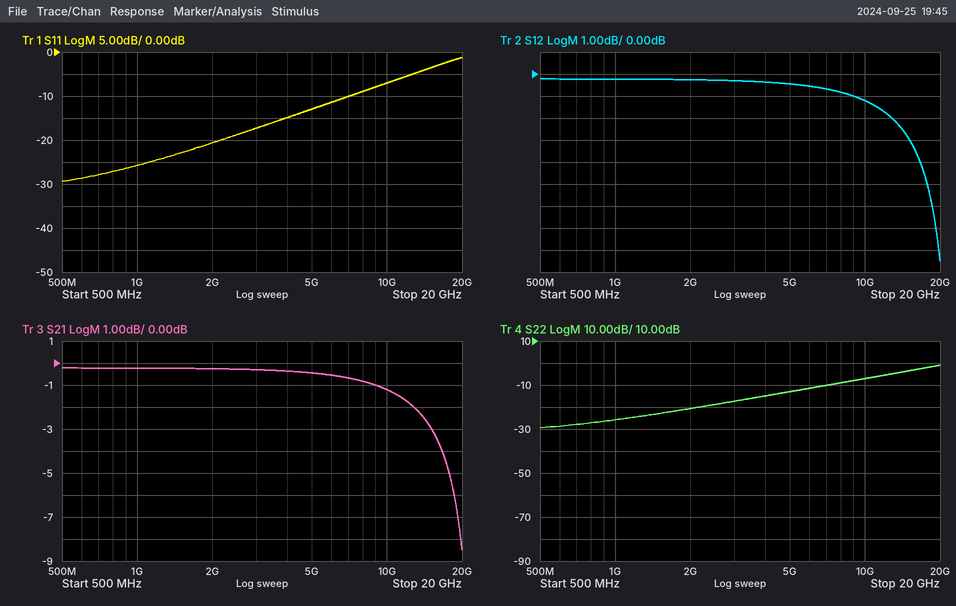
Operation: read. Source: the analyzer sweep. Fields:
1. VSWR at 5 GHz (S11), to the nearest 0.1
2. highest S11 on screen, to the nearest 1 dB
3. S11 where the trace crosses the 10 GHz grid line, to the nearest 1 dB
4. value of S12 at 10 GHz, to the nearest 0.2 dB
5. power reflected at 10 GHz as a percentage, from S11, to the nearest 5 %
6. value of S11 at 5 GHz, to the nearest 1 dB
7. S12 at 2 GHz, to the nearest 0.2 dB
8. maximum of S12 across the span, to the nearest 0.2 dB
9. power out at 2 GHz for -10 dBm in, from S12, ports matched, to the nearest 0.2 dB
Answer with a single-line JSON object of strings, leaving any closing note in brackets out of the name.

{"VSWR at 5 GHz (S11), to the nearest 0.1": "1.6", "highest S11 on screen, to the nearest 1 dB": "-1 dB", "S11 where the trace crosses the 10 GHz grid line, to the nearest 1 dB": "-7 dB", "value of S12 at 10 GHz, to the nearest 0.2 dB": "-1.2 dB", "power reflected at 10 GHz as a percentage, from S11, to the nearest 5 %": "20 %", "value of S11 at 5 GHz, to the nearest 1 dB": "-13 dB", "S12 at 2 GHz, to the nearest 0.2 dB": "-0.2 dB", "maximum of S12 across the span, to the nearest 0.2 dB": "-0.2 dB", "power out at 2 GHz for -10 dBm in, from S12, ports matched, to the nearest 0.2 dB": "-10.2 dBm"}
